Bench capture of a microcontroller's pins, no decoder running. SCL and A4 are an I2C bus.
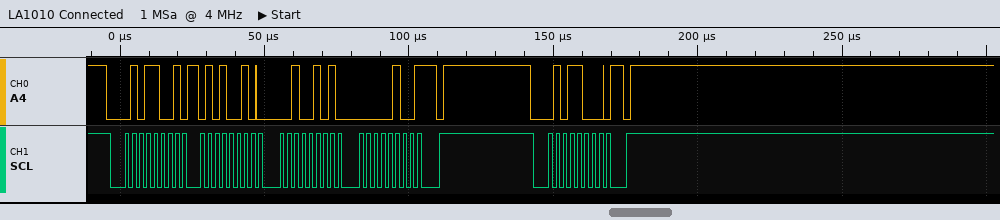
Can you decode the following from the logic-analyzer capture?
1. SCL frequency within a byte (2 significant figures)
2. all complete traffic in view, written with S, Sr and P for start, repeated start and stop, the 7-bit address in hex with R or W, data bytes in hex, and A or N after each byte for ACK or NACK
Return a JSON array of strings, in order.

["400 kHz", "S 2CR A 52 A 25 A 04 N P S 2CW A P"]
